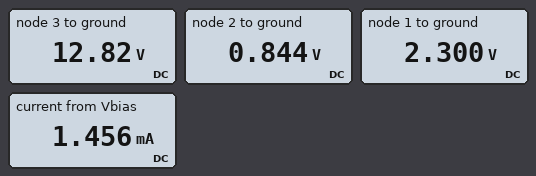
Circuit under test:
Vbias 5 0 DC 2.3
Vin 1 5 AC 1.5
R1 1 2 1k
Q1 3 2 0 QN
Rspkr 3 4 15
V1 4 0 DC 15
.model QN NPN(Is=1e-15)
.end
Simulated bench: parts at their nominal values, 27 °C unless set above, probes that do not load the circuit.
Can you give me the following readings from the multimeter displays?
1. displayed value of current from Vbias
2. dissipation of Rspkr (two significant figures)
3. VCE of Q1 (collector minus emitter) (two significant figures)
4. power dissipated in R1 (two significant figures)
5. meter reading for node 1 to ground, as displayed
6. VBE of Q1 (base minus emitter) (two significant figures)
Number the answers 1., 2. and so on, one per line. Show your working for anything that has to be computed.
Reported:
1. 1.456 mA
2. (15 V - 12.82 V)^2 / 15 Ω = 320 mW
3. 12.82 V = 13 V
4. (2.3 V - 844 mV)^2 / 1 kΩ = 2.1 mW
5. 2.300 V
6. 844 mV = 840 mV
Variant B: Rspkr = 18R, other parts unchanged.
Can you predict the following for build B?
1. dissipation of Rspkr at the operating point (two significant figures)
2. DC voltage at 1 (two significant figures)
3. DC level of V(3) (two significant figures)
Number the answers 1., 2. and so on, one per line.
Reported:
1. 380 mW
2. 2.3 V
3. 12 V
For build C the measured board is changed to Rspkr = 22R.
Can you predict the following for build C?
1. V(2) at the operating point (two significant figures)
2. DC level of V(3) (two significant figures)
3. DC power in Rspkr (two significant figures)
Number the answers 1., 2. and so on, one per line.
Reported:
1. 840 mV
2. 12 V
3. 470 mW
